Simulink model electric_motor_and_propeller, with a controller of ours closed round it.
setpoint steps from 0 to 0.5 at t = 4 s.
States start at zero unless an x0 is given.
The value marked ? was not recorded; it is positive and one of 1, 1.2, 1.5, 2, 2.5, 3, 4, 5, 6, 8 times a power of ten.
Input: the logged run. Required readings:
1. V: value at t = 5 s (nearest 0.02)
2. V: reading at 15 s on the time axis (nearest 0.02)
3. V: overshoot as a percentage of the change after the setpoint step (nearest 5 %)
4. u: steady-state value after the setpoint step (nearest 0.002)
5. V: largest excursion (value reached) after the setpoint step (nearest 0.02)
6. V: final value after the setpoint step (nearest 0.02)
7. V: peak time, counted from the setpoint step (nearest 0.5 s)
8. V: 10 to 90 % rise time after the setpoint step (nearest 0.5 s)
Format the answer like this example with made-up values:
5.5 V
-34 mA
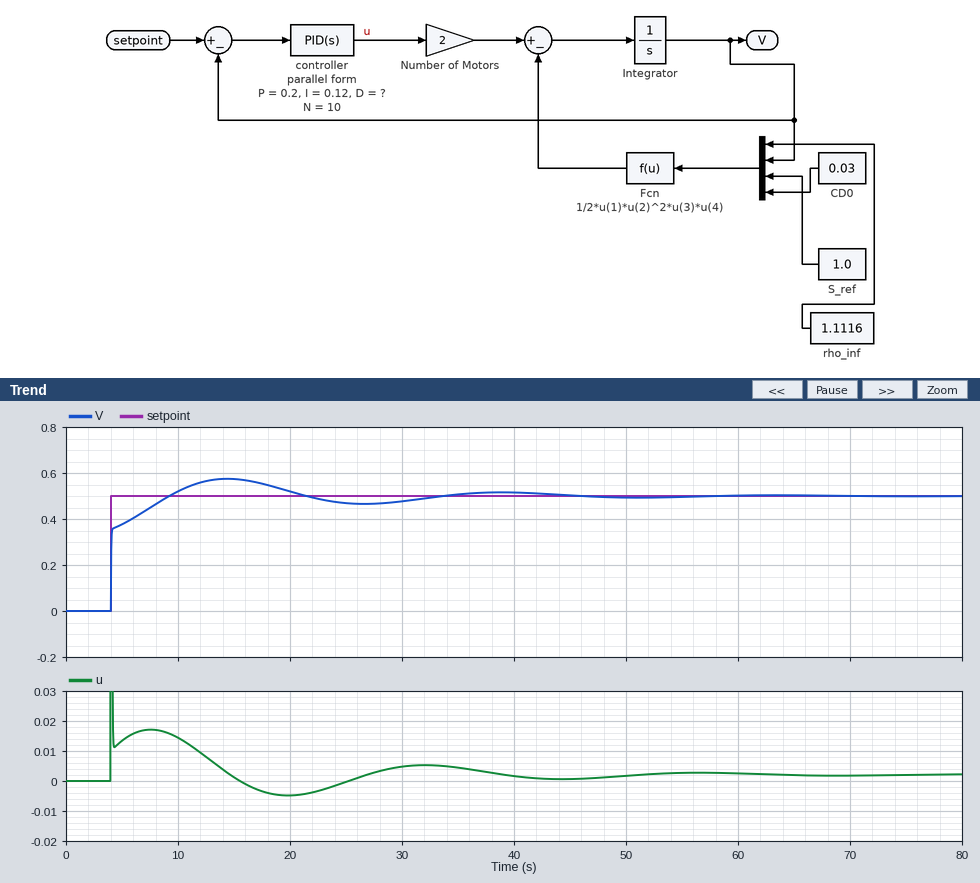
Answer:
0.38
0.58
15 %
0.002
0.58
0.50
10.5 s
3.5 s
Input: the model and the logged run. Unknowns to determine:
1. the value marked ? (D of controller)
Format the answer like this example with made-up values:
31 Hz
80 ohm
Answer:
1.2
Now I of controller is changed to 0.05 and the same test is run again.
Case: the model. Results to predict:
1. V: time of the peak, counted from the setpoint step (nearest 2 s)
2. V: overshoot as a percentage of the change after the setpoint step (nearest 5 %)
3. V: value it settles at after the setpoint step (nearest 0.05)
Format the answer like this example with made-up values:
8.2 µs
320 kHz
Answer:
16 s
10 %
0.50
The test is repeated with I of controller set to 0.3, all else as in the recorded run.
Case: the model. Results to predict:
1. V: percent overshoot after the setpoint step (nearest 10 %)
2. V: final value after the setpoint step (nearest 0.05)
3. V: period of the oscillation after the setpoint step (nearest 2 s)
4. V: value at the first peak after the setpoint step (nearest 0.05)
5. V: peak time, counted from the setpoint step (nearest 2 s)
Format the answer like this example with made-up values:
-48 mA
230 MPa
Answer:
20 %
0.50
16 s
0.60
6 s
